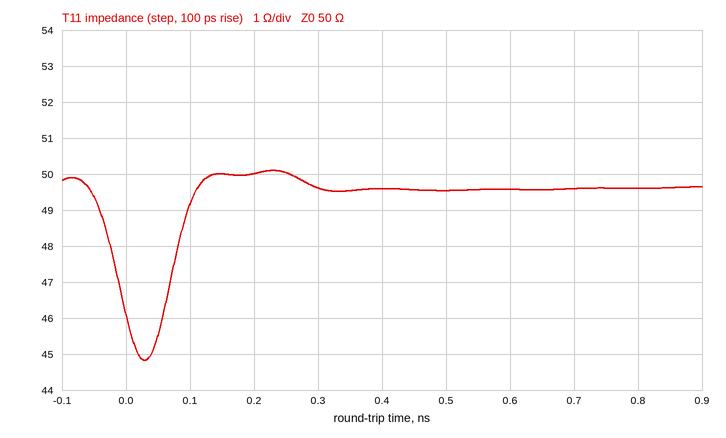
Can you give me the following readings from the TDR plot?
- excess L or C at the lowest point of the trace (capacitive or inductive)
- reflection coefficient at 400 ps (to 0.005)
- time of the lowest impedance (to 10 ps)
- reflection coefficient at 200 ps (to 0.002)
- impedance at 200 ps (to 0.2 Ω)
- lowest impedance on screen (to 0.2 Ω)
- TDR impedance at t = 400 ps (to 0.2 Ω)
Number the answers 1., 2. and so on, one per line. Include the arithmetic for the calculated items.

1. capacitive
2. (49.6 − 50)/(49.6 + 50) ≈ -0.00402, so -0.005 to the nearest 0.005
3. 30 ps
4. (50 − 50)/(50 + 50) ≈ 0.000
5. 50.0 Ω
6. 44.8 Ω
7. 49.6 Ω
